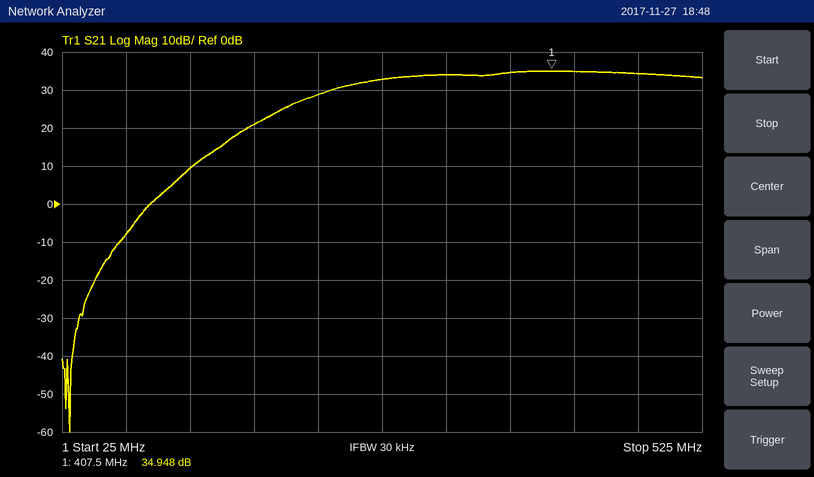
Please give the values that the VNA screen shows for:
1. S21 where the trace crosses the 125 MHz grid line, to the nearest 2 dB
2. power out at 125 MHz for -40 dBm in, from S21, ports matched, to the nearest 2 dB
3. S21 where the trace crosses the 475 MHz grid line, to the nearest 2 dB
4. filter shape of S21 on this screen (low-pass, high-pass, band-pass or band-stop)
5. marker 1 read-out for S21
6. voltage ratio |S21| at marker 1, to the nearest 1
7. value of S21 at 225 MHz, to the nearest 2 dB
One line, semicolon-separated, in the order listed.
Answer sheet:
10 dB; -30 dBm; 34 dB; high-pass; 34.948 dB; 56; 28 dB
